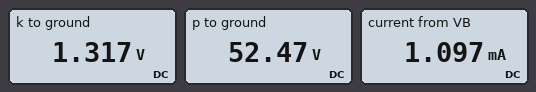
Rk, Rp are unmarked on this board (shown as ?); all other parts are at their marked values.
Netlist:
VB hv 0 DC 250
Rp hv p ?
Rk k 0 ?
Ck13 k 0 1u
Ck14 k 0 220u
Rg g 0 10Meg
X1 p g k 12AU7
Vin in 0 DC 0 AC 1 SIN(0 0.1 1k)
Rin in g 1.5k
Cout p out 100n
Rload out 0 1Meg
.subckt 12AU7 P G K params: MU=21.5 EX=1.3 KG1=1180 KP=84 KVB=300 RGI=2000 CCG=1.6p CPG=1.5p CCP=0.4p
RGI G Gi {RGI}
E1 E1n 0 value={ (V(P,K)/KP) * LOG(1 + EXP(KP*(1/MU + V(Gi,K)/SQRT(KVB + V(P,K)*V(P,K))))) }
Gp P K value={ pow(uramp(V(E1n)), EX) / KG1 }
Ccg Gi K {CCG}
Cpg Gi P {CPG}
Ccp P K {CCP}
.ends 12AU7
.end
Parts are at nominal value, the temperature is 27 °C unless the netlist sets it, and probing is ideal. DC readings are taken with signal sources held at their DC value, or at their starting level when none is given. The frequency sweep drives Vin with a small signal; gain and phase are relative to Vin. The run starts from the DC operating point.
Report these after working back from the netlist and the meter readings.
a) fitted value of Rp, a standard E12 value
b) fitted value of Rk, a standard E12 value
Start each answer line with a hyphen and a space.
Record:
- 180 kΩ
- 1.2 kΩ
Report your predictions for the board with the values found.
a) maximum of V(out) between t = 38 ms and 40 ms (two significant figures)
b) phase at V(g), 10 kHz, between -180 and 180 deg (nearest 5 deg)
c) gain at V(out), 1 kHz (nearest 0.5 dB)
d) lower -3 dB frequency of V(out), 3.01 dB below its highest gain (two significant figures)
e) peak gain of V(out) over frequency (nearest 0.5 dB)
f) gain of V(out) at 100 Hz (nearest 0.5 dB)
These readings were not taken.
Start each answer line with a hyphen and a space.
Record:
- 1.7 V
- 0 deg
- 24.5 dB
- 1.6 Hz
- 24.5 dB
- 24.5 dB
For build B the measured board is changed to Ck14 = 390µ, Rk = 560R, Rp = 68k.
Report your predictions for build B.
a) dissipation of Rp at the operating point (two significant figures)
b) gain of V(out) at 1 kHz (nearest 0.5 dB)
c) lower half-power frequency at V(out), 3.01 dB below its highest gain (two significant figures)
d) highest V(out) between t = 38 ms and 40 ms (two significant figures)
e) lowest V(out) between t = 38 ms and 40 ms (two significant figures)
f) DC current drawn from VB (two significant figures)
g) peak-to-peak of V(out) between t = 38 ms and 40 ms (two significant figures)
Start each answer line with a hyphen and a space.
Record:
- 430 mW
- 24.0 dB
- 1.7 Hz
- 1.6 V
- -1.6 V
- 2.5 mA
- 3.2 V
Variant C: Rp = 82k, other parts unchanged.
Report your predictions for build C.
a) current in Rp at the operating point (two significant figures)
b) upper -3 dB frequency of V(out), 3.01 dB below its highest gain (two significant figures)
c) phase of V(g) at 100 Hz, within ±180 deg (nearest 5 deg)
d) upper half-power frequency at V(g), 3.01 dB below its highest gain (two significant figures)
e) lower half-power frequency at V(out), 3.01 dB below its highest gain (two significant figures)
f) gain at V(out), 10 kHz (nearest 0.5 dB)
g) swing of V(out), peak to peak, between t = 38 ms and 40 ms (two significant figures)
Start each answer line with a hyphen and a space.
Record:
- 2.0 mA
- 1.4 MHz
- 0 deg
- 4.0 MHz
- 1.7 Hz
- 24.0 dB
- 3.1 V
